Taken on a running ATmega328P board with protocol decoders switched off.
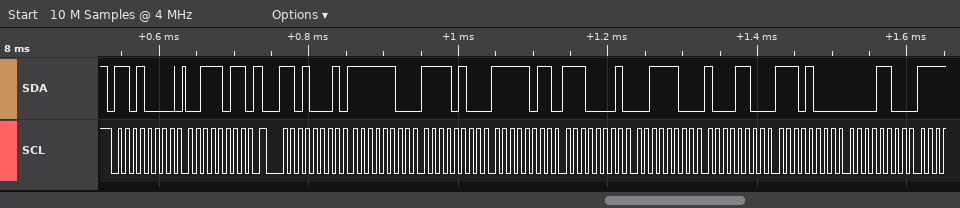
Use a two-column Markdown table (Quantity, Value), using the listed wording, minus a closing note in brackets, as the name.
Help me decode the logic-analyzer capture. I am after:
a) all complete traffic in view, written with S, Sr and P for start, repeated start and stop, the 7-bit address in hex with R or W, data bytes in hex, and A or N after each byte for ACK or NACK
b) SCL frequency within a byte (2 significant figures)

| Quantity | Value |
|---|---|
| all complete traffic in view, written with S, Sr and P for start, repeated start and stop, the 7-bit address in hex with R or W, data bytes in hex, and A or N after each byte for ACK or NACK | S 68W A 3B A Sr 68R A FC A F4 A FB A E1 A 3C A 8C A E8 A 0C A |
| SCL frequency within a byte | 100 kHz |
